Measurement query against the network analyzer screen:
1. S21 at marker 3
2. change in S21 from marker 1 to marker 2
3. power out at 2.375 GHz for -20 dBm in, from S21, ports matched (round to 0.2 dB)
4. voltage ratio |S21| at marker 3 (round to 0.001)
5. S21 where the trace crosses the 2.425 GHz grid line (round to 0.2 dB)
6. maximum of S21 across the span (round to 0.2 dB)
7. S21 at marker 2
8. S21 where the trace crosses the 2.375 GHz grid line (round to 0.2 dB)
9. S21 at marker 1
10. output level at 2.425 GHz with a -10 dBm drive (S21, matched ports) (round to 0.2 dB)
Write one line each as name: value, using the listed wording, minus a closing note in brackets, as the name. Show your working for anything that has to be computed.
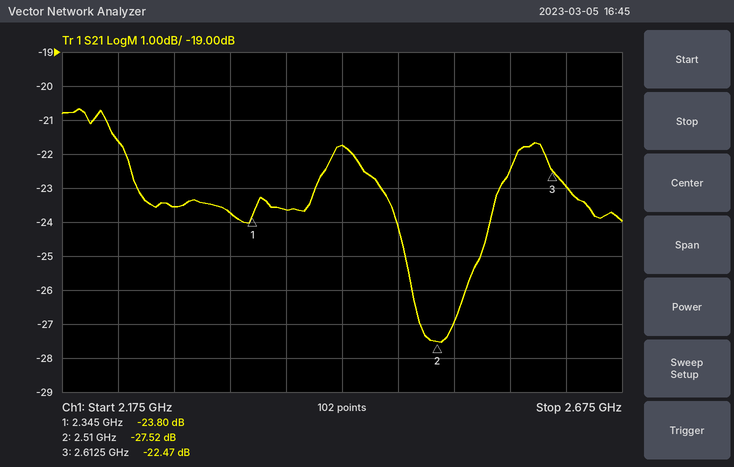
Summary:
S21 at marker 3: -22.47 dB
change in S21 from marker 1 to marker 2: -27.52 − (-23.8) = -3.72 dB
power out at 2.375 GHz for -20 dBm in, from S21, ports matched: -20 dBm + (-23.6 dB) = -43.6 dBm
voltage ratio |S21| at marker 3: 10^(-22.47/20) ≈ 0.075
S21 where the trace crosses the 2.425 GHz grid line: -21.8 dB
maximum of S21 across the span: -20.6 dB
S21 at marker 2: -27.52 dB
S21 where the trace crosses the 2.375 GHz grid line: -23.6 dB
S21 at marker 1: -23.80 dB
output level at 2.425 GHz with a -10 dBm drive (S21, matched ports): -10 dBm + (-21.8 dB) = -31.8 dBm
